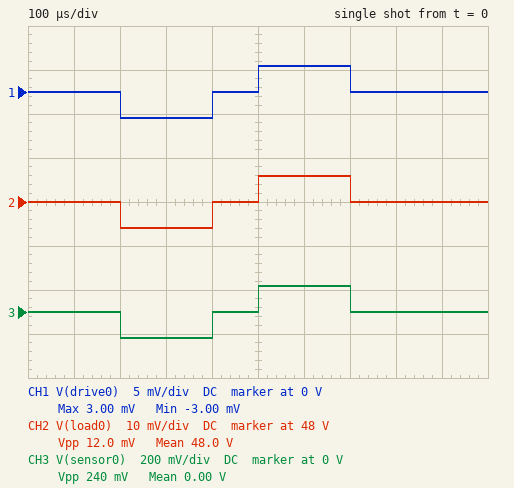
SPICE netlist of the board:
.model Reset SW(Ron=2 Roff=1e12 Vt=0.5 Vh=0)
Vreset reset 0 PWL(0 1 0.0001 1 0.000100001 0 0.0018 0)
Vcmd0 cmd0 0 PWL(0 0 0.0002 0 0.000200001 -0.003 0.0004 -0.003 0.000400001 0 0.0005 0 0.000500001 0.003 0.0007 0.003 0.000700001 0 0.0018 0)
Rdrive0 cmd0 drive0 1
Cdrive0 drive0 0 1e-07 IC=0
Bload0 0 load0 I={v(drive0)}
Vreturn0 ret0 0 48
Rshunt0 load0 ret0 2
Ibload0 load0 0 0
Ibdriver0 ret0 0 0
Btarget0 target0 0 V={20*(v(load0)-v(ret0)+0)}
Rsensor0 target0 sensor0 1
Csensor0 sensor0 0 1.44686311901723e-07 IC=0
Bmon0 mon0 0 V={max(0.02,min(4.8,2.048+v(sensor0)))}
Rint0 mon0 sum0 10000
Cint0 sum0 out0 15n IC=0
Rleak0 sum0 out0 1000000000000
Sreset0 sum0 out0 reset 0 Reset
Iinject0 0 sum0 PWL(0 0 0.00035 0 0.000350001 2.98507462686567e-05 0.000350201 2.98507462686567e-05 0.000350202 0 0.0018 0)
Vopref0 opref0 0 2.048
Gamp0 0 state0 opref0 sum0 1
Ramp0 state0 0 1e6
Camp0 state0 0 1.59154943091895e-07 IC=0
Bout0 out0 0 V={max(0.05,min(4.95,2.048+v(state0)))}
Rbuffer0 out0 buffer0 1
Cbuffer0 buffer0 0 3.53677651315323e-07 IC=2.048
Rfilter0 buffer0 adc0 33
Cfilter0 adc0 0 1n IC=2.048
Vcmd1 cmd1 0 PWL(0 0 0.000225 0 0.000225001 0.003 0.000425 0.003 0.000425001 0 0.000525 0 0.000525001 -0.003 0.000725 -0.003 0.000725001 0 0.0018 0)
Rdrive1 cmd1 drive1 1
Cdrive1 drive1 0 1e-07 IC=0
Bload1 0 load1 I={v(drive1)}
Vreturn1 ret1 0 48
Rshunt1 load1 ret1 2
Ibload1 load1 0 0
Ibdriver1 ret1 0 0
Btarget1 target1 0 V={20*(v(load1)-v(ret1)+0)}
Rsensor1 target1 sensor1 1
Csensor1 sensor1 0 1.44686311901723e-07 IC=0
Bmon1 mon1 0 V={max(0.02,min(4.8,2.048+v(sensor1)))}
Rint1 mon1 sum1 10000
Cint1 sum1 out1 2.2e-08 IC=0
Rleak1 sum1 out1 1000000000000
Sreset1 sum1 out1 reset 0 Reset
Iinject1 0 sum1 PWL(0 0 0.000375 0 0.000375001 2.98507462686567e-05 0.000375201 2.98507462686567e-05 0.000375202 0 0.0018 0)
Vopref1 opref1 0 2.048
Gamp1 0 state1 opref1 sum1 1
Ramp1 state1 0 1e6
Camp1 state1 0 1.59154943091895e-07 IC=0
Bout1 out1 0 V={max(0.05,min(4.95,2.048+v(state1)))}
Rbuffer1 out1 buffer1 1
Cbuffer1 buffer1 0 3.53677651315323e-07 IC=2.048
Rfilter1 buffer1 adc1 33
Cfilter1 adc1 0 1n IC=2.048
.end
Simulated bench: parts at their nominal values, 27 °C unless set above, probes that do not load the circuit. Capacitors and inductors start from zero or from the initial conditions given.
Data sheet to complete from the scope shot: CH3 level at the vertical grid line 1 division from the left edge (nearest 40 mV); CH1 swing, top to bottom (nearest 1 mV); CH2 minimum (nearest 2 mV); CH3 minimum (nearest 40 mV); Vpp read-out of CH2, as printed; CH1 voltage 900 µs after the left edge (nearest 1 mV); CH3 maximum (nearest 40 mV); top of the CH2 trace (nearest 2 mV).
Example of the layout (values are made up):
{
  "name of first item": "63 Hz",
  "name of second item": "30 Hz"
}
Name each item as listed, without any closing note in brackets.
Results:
{
  "CH3 level at the vertical grid line 1 division from the left edge": "0 V",
  "CH1 swing, top to bottom": "6 mV",
  "CH2 minimum": "47.994 V",
  "CH3 minimum": "-120 mV",
  "Vpp read-out of CH2, as printed": "12.0 mV",
  "CH1 voltage 900 µs after the left edge": "0 V",
  "CH3 maximum": "120 mV",
  "top of the CH2 trace": "48.006 V"
}
